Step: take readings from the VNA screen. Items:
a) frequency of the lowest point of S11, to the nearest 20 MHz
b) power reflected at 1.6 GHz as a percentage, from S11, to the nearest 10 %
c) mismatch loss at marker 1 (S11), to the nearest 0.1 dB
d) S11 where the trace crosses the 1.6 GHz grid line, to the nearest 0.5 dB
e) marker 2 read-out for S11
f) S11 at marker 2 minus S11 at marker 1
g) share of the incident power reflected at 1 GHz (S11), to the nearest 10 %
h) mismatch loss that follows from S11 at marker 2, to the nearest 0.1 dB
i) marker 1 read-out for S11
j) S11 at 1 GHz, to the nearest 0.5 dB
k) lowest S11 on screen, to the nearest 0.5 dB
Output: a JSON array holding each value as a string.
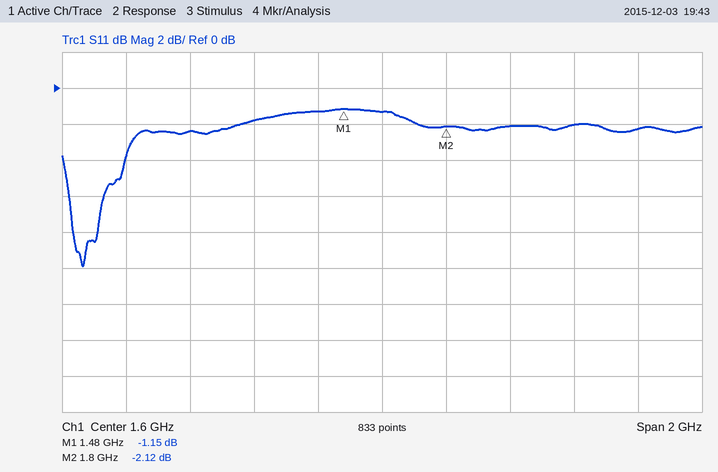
["660 MHz", "70 %", "6.3 dB", "-1.5 dB", "-2.12 dB", "-0.97 dB", "60 %", "4.1 dB", "-1.15 dB", "-2.5 dB", "-10.0 dB"]
